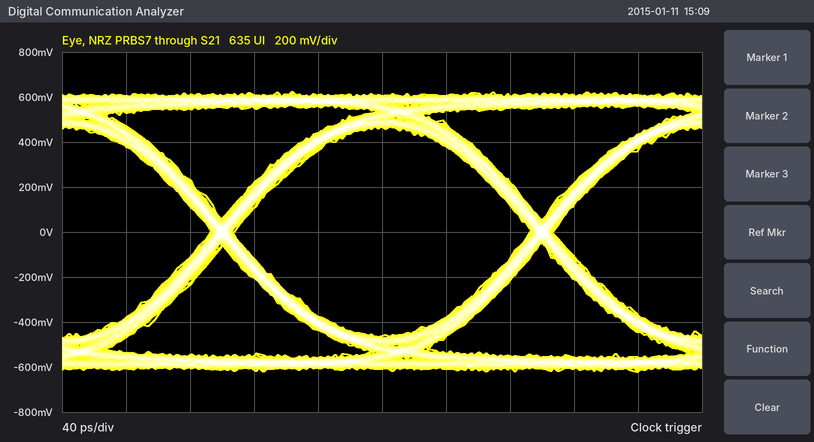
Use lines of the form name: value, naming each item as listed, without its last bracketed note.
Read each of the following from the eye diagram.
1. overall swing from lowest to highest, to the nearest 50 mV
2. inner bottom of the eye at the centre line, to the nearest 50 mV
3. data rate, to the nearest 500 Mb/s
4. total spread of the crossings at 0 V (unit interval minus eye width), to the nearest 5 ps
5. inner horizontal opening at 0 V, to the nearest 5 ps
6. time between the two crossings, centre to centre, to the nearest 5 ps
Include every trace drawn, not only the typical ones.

overall swing from lowest to highest, to the nearest 50 mV: 1.25 V
inner bottom of the eye at the centre line, to the nearest 50 mV: -450 mV
data rate, to the nearest 500 Mb/s: 5.0 Gb/s
total spread of the crossings at 0 V (unit interval minus eye width), to the nearest 5 ps: 15 ps
inner horizontal opening at 0 V, to the nearest 5 ps: 185 ps
time between the two crossings, centre to centre, to the nearest 5 ps: 200 ps
